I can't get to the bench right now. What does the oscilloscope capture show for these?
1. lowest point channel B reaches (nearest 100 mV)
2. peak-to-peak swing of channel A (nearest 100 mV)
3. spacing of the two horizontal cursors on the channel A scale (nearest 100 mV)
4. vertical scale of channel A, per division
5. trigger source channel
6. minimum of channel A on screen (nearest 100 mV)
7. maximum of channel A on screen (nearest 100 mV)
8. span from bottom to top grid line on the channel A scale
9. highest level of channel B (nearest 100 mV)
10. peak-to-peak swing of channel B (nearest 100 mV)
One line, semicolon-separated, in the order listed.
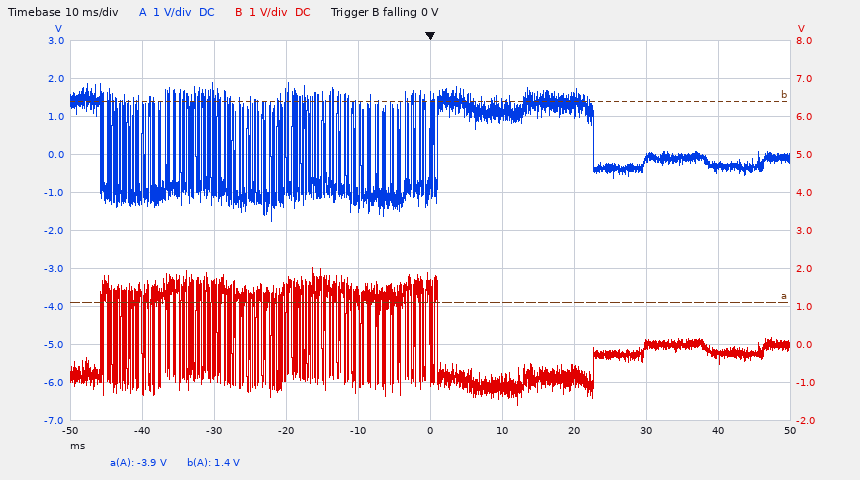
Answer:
-1.6 V; 3.7 V; 5.3 V; 1 V; channel B; -1.8 V; 1.9 V; 10 V; 2.0 V; 3.6 V
